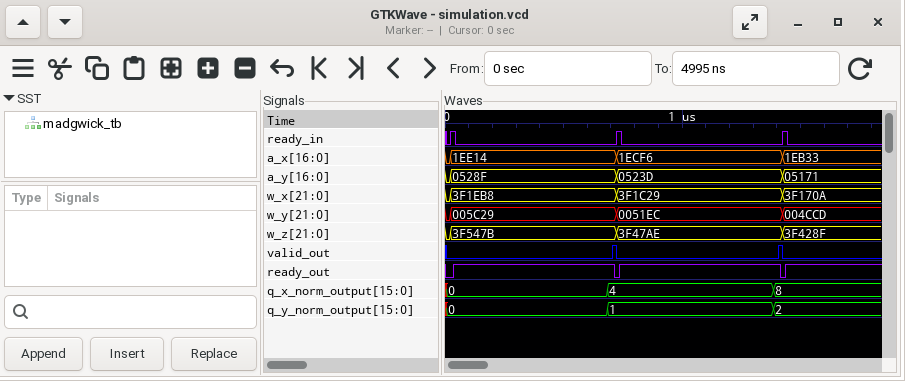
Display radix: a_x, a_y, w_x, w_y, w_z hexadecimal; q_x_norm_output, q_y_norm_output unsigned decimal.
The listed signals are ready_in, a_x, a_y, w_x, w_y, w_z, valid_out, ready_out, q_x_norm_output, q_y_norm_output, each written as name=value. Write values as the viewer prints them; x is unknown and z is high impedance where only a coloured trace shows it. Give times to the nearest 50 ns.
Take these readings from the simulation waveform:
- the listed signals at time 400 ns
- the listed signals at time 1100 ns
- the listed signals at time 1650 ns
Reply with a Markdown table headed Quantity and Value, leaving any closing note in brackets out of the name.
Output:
| Quantity | Value |
|---|---|
| the listed signals at time 400 ns | ready_in=0, a_x=1EE14, a_y=0528F, w_x=3F1EB8, w_y=005C29, w_z=3F547B, valid_out=0, ready_out=1, q_x_norm_output=0, q_y_norm_output=0 |
| the listed signals at time 1100 ns | ready_in=0, a_x=1ECF6, a_y=0523D, w_x=3F1C29, w_y=0051EC, w_z=3F47AE, valid_out=0, ready_out=1, q_x_norm_output=4, q_y_norm_output=1 |
| the listed signals at time 1650 ns | ready_in=0, a_x=1EB33, a_y=05171, w_x=3F170A, w_y=004CCD, w_z=3F428F, valid_out=0, ready_out=1, q_x_norm_output=8, q_y_norm_output=2 |
